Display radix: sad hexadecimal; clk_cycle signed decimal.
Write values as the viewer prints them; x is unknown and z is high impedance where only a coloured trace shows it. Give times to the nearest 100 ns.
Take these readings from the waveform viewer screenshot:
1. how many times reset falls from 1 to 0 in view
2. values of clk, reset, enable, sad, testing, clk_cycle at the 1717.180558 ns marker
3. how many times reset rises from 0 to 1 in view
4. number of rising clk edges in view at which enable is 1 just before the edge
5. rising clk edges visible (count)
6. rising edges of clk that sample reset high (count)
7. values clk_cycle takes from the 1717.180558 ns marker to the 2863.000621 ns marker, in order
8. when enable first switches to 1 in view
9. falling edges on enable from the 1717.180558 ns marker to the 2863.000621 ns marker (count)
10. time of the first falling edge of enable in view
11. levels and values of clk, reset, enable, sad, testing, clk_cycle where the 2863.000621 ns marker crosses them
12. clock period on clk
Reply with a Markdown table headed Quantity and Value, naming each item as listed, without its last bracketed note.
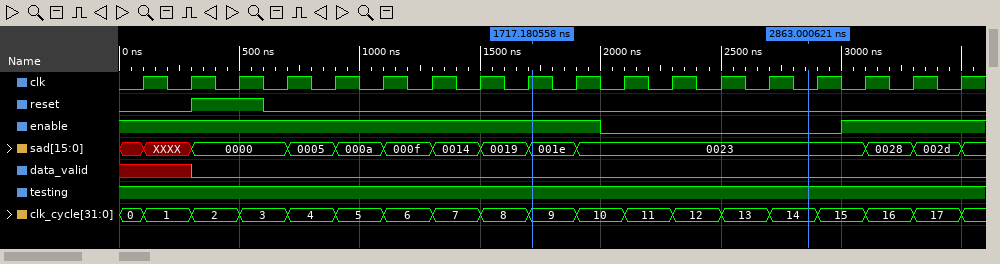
| Quantity | Value |
|---|---|
| how many times reset falls from 1 to 0 in view | 1 |
| values of clk, reset, enable, sad, testing, clk_cycle at the 1717.180558 ns marker | clk=1, reset=0, enable=1, sad=001e, testing=1, clk_cycle=9 |
| how many times reset rises from 0 to 1 in view | 1 |
| number of rising clk edges in view at which enable is 1 just before the edge | 13 |
| rising clk edges visible | 18 |
| rising edges of clk that sample reset high | 1 |
| values clk_cycle takes from the 1717.180558 ns marker to the 2863.000621 ns marker, in order | 9, 10, 11, 12, 13, 14 |
| when enable first switches to 1 in view | 3000 ns |
| falling edges on enable from the 1717.180558 ns marker to the 2863.000621 ns marker | 1 |
| time of the first falling edge of enable in view | 2000 ns |
| levels and values of clk, reset, enable, sad, testing, clk_cycle where the 2863.000621 ns marker crosses them | clk=0, reset=0, enable=0, sad=0023, testing=1, clk_cycle=14 |
| clock period on clk | 200 ns |
